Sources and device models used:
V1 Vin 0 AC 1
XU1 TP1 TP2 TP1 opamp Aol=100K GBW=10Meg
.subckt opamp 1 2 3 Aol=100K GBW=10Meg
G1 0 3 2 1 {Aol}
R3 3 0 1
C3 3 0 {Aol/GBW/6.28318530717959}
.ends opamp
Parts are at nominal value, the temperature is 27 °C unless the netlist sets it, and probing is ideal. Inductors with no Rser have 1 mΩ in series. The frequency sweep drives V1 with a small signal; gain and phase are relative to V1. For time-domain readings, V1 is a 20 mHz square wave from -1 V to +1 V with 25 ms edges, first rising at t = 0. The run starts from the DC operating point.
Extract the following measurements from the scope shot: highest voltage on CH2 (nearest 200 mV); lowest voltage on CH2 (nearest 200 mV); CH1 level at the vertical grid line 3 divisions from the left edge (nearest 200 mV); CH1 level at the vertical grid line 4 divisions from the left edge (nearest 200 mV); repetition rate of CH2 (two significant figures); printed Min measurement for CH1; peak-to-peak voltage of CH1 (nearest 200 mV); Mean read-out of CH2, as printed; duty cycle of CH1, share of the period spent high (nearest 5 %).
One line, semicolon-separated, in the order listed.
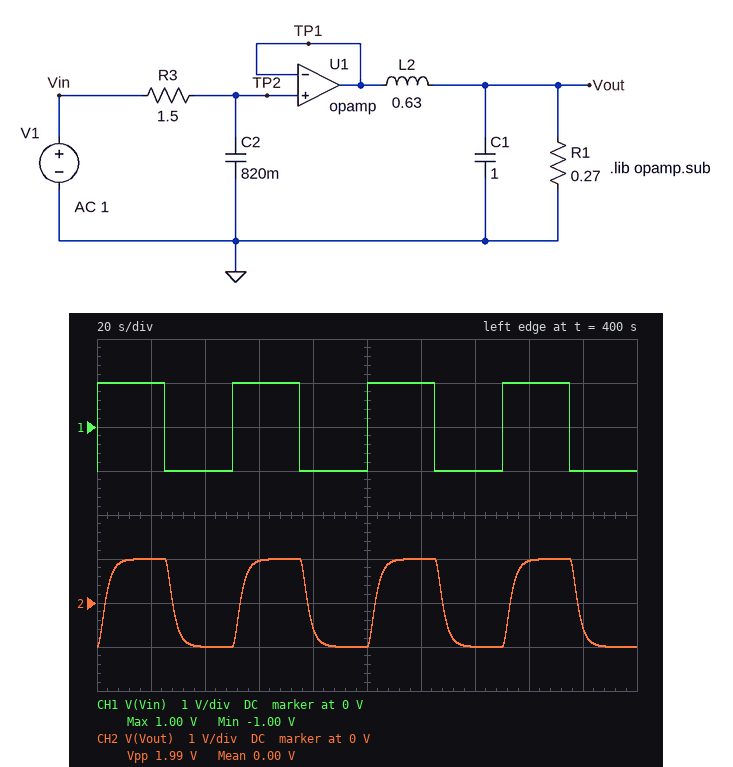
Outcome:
1.0 V; -1.0 V; 1.0 V; -1.0 V; 20 mHz; -1.00 V; 2.0 V; 0.00 V; 50 %
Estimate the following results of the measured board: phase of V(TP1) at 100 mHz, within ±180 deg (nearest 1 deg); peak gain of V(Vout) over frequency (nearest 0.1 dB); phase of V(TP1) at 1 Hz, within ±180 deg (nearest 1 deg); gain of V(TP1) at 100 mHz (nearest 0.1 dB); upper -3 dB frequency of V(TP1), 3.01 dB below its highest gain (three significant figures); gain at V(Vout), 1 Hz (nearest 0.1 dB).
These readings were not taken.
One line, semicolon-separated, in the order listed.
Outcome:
-38 deg; 0 dB; -83 deg; -2.0 dB; 129 mHz; -46.8 dB
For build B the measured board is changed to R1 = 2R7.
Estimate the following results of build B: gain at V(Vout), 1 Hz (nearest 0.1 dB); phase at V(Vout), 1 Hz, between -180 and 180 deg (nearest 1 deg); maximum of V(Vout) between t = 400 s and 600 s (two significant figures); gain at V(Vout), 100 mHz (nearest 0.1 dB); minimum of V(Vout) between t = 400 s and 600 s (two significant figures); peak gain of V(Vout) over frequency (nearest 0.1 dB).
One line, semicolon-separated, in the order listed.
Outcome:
-45.4 dB; 101 deg; 1.5 V; 0.3 dB; -1.5 V; 5.6 dB
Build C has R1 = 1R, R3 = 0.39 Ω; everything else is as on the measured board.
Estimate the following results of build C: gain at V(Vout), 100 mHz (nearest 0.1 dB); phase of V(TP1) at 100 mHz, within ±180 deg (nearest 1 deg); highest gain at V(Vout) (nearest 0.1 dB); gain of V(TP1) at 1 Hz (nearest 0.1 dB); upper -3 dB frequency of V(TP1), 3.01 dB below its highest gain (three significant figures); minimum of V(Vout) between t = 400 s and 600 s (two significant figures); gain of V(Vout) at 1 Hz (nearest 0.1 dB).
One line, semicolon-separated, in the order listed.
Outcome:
1.2 dB; -11 deg; 2.3 dB; -7.0 dB; 498 mHz; -1.5 V; -34.7 dB
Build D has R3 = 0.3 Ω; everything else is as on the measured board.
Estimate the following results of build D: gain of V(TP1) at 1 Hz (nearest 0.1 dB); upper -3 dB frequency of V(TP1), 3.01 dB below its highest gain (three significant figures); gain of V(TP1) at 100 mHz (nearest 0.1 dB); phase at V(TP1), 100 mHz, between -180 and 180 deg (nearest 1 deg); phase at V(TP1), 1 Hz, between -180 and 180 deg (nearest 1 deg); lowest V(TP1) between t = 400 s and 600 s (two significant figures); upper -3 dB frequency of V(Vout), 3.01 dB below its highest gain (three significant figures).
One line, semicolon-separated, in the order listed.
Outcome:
-5.3 dB; 647 mHz; -0.1 dB; -9 deg; -57 deg; -1.0 V; 76.2 mHz
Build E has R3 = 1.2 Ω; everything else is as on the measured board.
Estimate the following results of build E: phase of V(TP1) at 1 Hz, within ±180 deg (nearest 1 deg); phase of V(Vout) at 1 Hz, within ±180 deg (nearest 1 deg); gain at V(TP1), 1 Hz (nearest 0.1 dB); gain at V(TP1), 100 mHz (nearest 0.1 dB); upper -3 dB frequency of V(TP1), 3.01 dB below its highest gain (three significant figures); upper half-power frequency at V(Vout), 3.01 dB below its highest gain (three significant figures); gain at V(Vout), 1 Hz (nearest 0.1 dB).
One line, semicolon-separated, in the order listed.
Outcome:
-81 deg; 131 deg; -15.9 dB; -1.4 dB; 162 mHz; 65.6 mHz; -44.9 dB
